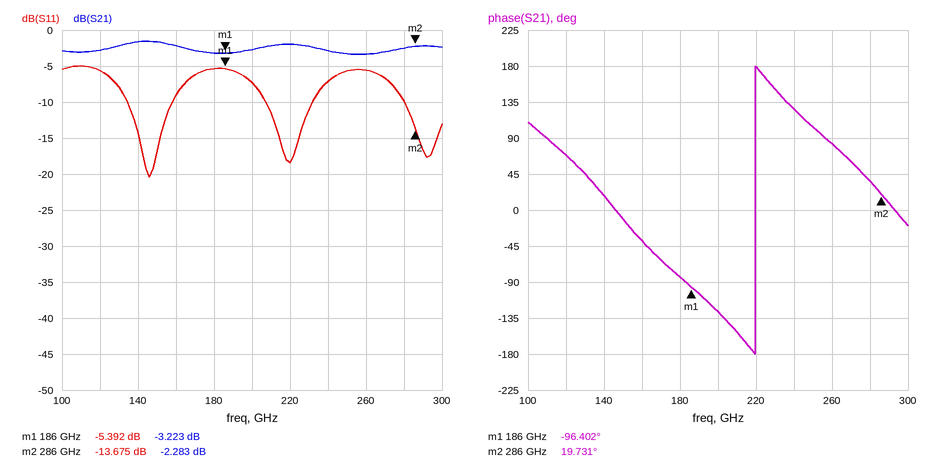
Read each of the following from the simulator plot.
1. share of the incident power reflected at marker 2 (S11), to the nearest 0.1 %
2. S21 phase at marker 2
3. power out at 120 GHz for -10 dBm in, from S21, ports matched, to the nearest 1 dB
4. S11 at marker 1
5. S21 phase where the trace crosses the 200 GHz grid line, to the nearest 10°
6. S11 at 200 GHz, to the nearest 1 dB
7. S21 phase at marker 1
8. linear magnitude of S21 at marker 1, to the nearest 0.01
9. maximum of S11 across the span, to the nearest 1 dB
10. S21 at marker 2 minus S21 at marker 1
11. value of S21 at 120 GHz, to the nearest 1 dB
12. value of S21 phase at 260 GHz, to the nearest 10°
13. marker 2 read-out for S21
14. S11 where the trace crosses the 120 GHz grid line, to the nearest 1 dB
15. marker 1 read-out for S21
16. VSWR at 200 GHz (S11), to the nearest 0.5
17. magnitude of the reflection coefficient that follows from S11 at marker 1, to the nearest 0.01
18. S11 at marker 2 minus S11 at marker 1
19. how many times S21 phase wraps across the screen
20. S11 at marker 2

4.3 %
19.731°
-13 dBm
-5.392 dB
-130°
-7 dB
-96.402°
0.69
-5 dB
0.940 dB
-3 dB
80°
-2.283 dB
-6 dB
-3.223 dB
2.5
0.54
-8.283 dB
1
-13.675 dB
